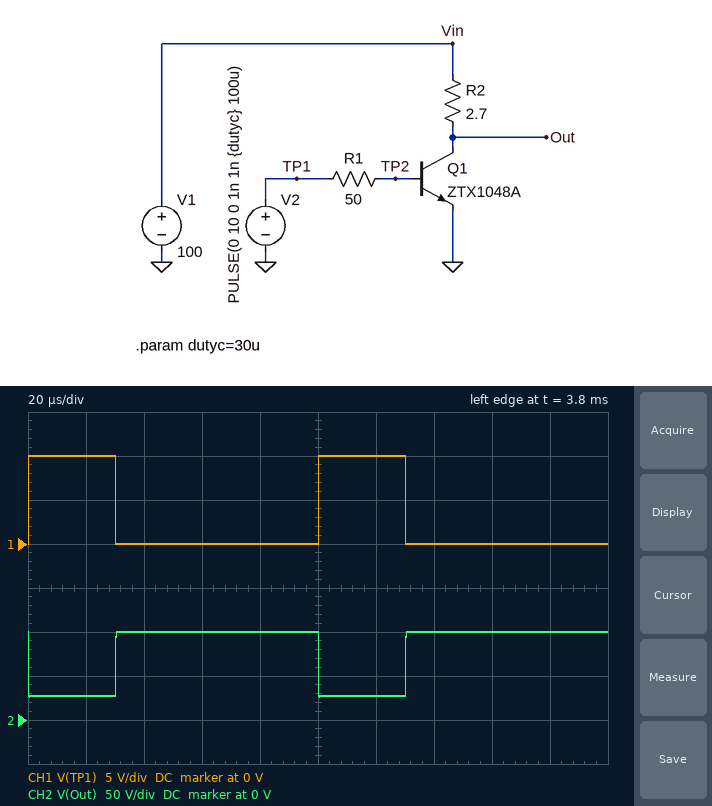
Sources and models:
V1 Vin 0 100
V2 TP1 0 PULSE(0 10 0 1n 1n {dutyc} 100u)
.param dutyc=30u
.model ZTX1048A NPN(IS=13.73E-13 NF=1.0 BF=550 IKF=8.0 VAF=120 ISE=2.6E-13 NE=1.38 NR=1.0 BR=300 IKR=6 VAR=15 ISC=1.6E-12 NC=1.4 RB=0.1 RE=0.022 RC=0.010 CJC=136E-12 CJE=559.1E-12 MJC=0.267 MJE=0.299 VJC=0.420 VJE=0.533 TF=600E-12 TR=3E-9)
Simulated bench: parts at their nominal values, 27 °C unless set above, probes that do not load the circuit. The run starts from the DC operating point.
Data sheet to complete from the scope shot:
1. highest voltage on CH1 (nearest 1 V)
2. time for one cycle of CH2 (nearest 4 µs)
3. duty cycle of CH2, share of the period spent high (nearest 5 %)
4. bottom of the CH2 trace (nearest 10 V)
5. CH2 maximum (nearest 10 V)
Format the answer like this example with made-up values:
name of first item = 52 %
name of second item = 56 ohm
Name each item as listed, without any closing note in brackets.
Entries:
highest voltage on CH1 = 10 V
time for one cycle of CH2 = 100 µs
duty cycle of CH2, share of the period spent high = 70 %
bottom of the CH2 trace = 30 V
CH2 maximum = 100 V
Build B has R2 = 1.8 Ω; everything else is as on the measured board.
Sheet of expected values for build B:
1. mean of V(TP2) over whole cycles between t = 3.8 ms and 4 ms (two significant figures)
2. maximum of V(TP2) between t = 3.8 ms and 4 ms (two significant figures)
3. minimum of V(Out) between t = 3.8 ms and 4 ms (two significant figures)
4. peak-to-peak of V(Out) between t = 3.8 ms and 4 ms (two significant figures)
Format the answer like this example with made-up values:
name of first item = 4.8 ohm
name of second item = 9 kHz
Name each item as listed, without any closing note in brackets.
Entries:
mean of V(TP2) over whole cycles between t = 3.8 ms and 4 ms = 460 mV
maximum of V(TP2) between t = 3.8 ms and 4 ms = 1.5 V
minimum of V(Out) between t = 3.8 ms and 4 ms = 45 V
peak-to-peak of V(Out) between t = 3.8 ms and 4 ms = 55 V
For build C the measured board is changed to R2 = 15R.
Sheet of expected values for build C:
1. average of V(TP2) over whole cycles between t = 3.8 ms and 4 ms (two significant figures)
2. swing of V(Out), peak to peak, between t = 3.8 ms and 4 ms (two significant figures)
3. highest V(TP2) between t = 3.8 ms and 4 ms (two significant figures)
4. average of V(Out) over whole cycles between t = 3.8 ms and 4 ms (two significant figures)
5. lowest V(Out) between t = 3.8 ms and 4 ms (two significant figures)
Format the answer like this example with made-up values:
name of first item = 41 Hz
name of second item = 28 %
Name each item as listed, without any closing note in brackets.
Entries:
average of V(TP2) over whole cycles between t = 3.8 ms and 4 ms = 300 mV
swing of V(Out), peak to peak, between t = 3.8 ms and 4 ms = 100 V
highest V(TP2) between t = 3.8 ms and 4 ms = 980 mV
average of V(Out) over whole cycles between t = 3.8 ms and 4 ms = 69 V
lowest V(Out) between t = 3.8 ms and 4 ms = 230 mV
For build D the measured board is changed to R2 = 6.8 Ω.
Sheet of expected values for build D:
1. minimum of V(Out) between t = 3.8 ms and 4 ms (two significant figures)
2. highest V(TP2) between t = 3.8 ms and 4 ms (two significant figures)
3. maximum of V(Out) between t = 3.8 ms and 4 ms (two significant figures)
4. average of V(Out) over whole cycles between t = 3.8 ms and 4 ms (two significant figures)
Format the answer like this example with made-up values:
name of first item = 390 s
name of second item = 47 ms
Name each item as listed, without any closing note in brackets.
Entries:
minimum of V(Out) between t = 3.8 ms and 4 ms = 510 mV
highest V(TP2) between t = 3.8 ms and 4 ms = 1.2 V
maximum of V(Out) between t = 3.8 ms and 4 ms = 100 V
average of V(Out) over whole cycles between t = 3.8 ms and 4 ms = 70 V
